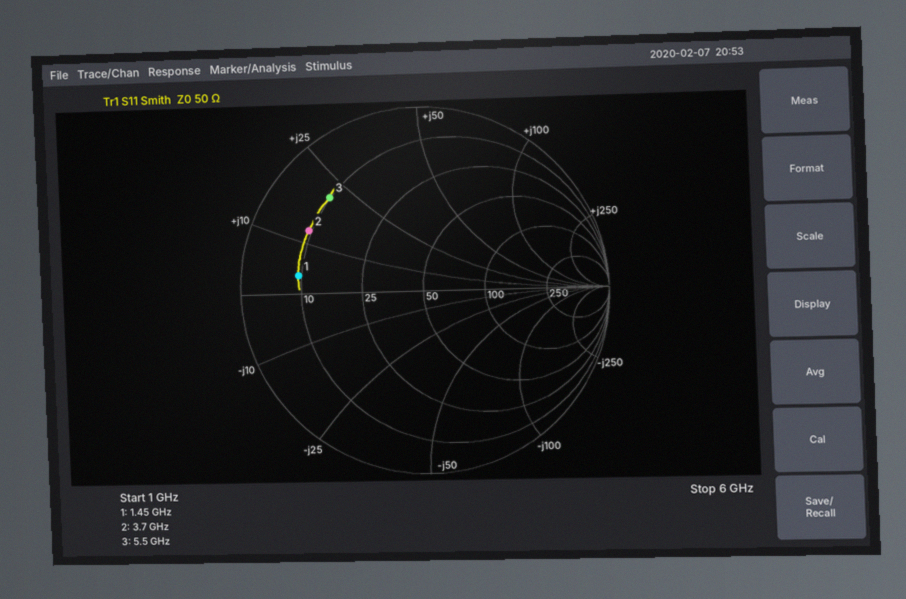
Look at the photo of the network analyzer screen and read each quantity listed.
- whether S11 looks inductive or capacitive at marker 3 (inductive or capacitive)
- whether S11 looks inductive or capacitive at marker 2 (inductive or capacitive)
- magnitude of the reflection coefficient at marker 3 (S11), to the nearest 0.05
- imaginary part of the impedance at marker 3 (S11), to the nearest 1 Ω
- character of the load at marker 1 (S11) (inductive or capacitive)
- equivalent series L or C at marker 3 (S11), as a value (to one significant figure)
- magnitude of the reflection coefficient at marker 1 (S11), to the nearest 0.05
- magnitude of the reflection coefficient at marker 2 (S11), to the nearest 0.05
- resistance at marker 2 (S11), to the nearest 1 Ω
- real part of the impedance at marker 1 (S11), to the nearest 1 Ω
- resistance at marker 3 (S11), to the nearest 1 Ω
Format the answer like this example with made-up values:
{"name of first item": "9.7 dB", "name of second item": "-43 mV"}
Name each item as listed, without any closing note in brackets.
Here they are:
{"whether S11 looks inductive or capacitive at marker 3": "inductive", "whether S11 looks inductive or capacitive at marker 2": "inductive", "magnitude of the reflection coefficient at marker 3 (S11), to the nearest 0.05": "0.70", "imaginary part of the impedance at marker 3 (S11), to the nearest 1 Ω": "+21 Ω", "character of the load at marker 1 (S11)": "inductive", "equivalent series L or C at marker 3 (S11), as a value": "600 pH", "magnitude of the reflection coefficient at marker 1 (S11), to the nearest 0.05": "0.70", "magnitude of the reflection coefficient at marker 2 (S11), to the nearest 0.05": "0.70", "resistance at marker 2 (S11), to the nearest 1 Ω": "9 Ω", "real part of the impedance at marker 1 (S11), to the nearest 1 Ω": "9 Ω", "resistance at marker 3 (S11), to the nearest 1 Ω": "10 Ω"}
